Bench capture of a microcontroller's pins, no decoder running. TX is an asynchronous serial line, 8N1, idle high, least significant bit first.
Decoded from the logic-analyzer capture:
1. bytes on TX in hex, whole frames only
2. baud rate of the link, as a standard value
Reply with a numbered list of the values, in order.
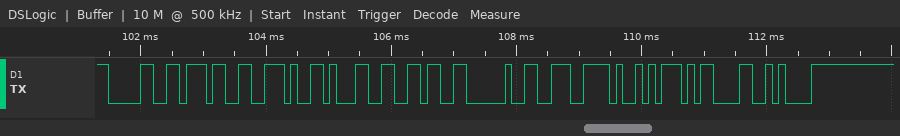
1. 0x30 0x37 0x2E 0x31 0x36 0x20 0xCE 0xA9 0x0D 0x0A
2. 9600 baud
